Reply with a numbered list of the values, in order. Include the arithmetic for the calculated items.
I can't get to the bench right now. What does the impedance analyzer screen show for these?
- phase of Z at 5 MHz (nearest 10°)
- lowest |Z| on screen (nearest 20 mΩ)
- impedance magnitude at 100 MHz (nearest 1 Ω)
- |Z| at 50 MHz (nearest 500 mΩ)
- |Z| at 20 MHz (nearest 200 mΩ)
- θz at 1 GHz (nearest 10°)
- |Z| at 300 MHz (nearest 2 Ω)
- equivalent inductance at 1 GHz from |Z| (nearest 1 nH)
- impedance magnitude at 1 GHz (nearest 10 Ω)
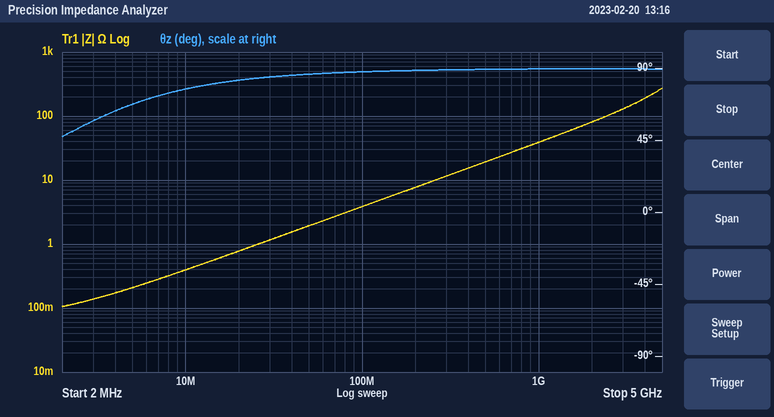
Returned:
1. 70°
2. 100 mΩ
3. 4 Ω
4. 2.0 Ω
5. 800 mΩ
6. 90°
7. 12 Ω
8. L = 40 Ω/(2π × 1 GHz) ≈ 6 nH
9. 40 Ω
